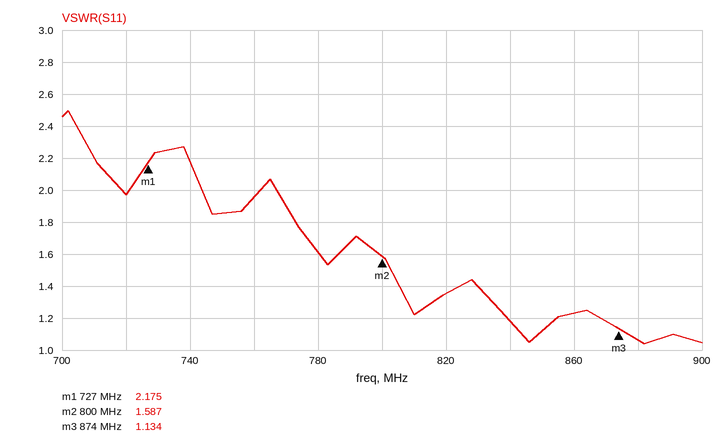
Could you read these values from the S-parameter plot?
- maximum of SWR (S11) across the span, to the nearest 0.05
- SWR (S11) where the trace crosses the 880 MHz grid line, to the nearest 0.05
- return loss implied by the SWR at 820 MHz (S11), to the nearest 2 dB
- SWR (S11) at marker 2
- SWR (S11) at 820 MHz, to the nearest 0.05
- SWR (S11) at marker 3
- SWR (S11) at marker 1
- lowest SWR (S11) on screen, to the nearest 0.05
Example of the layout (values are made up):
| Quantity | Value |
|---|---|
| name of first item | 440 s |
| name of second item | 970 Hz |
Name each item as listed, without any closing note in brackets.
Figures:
| Quantity | Value |
|---|---|
| maximum of SWR (S11) across the span, to the nearest 0.05 | 2.50 |
| SWR (S11) where the trace crosses the 880 MHz grid line, to the nearest 0.05 | 1.05 |
| return loss implied by the SWR at 820 MHz (S11), to the nearest 2 dB | 16 dB |
| SWR (S11) at marker 2 | 1.587 |
| SWR (S11) at 820 MHz, to the nearest 0.05 | 1.35 |
| SWR (S11) at marker 3 | 1.134 |
| SWR (S11) at marker 1 | 2.175 |
| lowest SWR (S11) on screen, to the nearest 0.05 | 1.05 |
